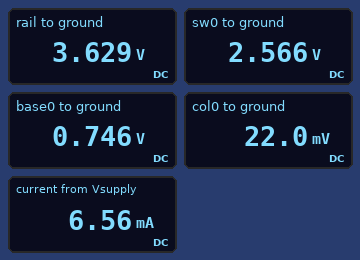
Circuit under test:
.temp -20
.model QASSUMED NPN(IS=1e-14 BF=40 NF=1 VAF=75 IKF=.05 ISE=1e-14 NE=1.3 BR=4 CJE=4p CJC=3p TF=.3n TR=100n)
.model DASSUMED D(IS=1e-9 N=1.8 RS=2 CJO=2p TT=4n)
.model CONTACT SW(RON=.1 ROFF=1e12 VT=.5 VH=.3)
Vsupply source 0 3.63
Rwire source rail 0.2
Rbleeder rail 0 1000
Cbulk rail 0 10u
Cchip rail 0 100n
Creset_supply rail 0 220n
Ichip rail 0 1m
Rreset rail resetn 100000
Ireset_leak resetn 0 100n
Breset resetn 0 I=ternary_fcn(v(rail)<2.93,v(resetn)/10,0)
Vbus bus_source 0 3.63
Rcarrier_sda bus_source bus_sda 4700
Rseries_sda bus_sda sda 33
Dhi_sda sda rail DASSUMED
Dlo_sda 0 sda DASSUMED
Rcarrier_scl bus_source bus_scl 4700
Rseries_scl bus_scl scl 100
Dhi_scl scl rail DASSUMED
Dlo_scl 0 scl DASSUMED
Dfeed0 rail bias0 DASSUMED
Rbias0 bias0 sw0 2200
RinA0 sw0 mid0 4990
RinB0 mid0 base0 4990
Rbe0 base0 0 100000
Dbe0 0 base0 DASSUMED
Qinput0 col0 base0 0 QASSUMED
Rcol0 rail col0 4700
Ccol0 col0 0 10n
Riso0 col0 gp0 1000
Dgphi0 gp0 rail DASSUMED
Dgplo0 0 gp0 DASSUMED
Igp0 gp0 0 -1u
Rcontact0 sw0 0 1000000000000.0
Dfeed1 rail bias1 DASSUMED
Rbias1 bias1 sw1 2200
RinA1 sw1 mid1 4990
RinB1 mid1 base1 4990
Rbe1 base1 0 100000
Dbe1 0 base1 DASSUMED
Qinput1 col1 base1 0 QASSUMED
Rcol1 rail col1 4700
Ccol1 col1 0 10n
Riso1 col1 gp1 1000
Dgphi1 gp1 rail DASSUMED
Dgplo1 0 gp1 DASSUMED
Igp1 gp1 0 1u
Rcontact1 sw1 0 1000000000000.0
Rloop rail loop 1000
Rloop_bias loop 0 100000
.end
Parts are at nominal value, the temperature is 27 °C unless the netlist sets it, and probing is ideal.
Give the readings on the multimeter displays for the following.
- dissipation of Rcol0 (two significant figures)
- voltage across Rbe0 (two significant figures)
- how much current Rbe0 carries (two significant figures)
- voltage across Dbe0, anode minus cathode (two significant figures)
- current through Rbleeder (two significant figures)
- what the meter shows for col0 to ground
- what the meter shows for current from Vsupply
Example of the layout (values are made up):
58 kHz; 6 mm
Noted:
2.8 mW; 750 mV; 7.5 µA; -750 mV; 3.6 mA; 22.0 mV; 6.56 mA
